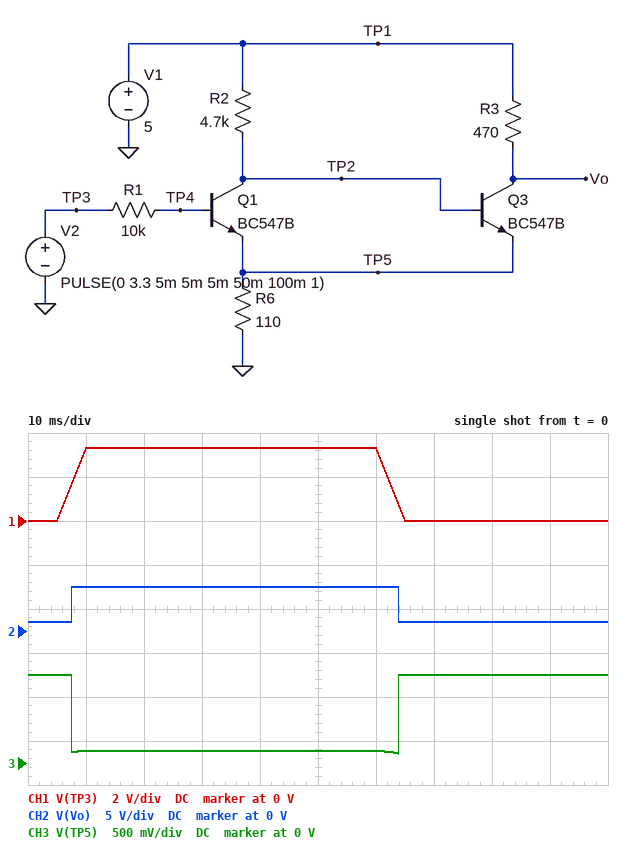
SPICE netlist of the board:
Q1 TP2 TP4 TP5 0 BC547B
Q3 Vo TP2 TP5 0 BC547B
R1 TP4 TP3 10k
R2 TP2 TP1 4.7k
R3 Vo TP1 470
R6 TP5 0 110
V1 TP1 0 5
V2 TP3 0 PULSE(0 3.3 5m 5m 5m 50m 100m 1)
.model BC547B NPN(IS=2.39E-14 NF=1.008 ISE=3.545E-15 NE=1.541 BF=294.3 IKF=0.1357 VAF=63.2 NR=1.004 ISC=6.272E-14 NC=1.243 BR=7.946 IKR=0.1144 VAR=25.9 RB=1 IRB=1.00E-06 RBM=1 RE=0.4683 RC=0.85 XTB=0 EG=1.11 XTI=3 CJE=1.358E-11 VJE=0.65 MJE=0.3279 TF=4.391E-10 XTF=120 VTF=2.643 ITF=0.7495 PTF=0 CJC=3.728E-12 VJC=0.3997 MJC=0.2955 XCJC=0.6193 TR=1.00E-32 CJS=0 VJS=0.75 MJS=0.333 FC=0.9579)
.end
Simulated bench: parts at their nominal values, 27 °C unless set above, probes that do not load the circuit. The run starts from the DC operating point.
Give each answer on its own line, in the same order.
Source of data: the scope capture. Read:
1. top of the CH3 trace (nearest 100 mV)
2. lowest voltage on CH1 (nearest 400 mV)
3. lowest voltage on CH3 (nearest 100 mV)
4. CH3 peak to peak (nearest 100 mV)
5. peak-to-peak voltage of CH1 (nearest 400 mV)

1.0 V
0 V
100 mV
900 mV
3.2 V
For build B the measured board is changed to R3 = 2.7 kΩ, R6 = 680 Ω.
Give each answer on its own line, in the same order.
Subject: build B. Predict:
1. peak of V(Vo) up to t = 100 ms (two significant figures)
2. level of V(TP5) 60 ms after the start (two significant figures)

5.0 V
740 mV
